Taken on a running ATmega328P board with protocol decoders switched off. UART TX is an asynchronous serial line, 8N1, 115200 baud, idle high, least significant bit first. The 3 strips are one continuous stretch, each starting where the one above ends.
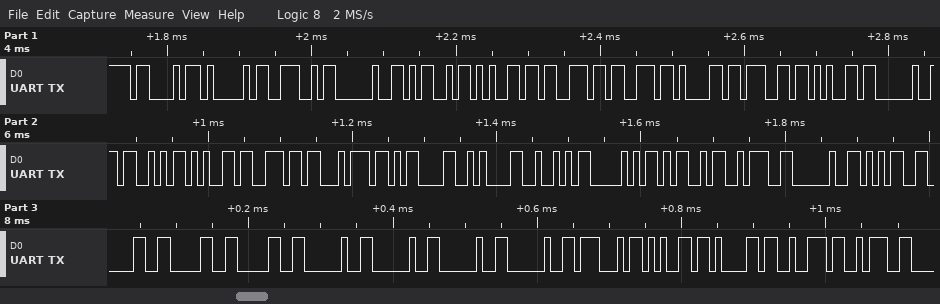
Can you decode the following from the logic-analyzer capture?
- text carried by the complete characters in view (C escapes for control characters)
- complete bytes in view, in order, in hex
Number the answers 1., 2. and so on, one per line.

1. "CAN Message Sent\r\nRPM: 5000    Gear:"
2. 43 41 4E 20 4D 65 73 73 61 67 65 20 53 65 6E 74 0D 0A 52 50 4D 3A 20 35 30 30 30 20 20 20 20 47 65 61 72 3A
